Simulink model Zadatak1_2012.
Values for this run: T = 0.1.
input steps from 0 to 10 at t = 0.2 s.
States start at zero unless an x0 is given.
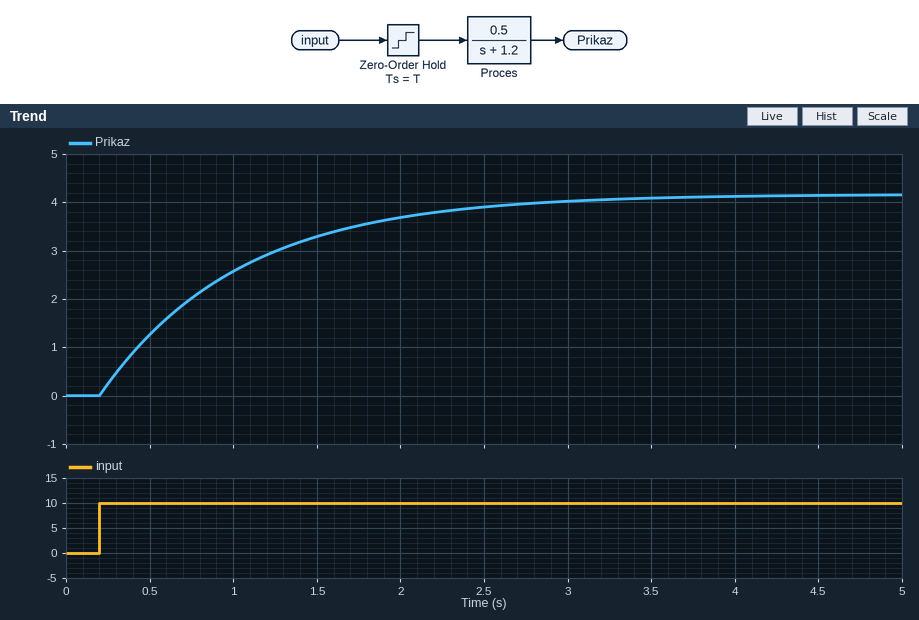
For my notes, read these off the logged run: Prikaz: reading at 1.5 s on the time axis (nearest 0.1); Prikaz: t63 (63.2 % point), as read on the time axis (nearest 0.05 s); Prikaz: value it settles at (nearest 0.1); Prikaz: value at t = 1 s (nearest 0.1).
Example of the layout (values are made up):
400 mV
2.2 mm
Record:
3.3
1.05 s
4.2
2.6
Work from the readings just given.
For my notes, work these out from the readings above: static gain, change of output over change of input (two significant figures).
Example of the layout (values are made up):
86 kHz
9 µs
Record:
0.42
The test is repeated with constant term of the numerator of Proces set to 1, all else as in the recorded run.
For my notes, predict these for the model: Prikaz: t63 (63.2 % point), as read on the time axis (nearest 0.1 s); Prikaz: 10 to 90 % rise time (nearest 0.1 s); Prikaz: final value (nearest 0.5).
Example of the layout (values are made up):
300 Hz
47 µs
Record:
1.0 s
1.8 s
8.5
